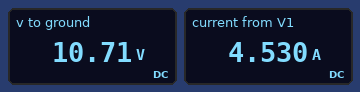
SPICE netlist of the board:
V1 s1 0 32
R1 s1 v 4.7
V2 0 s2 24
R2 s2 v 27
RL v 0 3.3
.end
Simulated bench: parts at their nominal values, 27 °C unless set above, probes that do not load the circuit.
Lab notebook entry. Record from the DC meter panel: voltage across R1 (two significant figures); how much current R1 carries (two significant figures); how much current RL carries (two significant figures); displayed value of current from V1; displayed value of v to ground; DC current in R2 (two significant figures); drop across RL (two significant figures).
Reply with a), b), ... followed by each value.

a) 21 V
b) 4.5 A
c) 3.2 A
d) 4.530 A
e) 10.71 V
f) 1.3 A
g) 11 V
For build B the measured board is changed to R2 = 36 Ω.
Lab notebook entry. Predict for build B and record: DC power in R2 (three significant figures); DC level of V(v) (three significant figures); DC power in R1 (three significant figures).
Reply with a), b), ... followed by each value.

a) 34.6 W
b) 11.3 V
c) 91.2 W
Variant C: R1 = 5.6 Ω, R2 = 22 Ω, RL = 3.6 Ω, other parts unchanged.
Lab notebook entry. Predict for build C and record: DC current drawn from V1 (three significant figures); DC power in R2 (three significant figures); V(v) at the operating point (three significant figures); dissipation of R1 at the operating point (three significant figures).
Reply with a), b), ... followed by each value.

a) 4.07 A
b) 50.1 W
c) 9.21 V
d) 92.7 W
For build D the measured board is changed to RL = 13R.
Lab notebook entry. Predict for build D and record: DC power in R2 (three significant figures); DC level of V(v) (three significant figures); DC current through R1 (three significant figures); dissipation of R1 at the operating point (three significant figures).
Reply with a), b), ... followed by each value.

a) 65.7 W
b) 18.1 V
c) 2.95 A
d) 41.0 W
